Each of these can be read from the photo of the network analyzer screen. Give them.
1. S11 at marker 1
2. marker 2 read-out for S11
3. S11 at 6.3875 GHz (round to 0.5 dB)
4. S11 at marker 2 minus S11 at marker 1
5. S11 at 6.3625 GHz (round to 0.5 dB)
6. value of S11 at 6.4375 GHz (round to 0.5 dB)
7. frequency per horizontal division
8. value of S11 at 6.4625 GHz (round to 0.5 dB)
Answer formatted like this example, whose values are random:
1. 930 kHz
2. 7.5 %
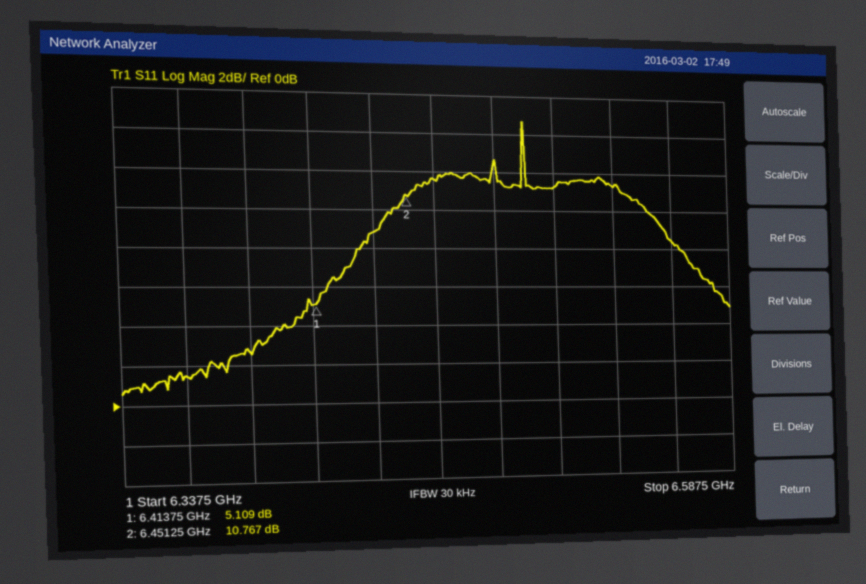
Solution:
1. 5.109 dB
2. 10.767 dB
3. 2.5 dB
4. 5.658 dB
5. 1.5 dB
6. 9.0 dB
7. 25 MHz
8. 11.5 dB
